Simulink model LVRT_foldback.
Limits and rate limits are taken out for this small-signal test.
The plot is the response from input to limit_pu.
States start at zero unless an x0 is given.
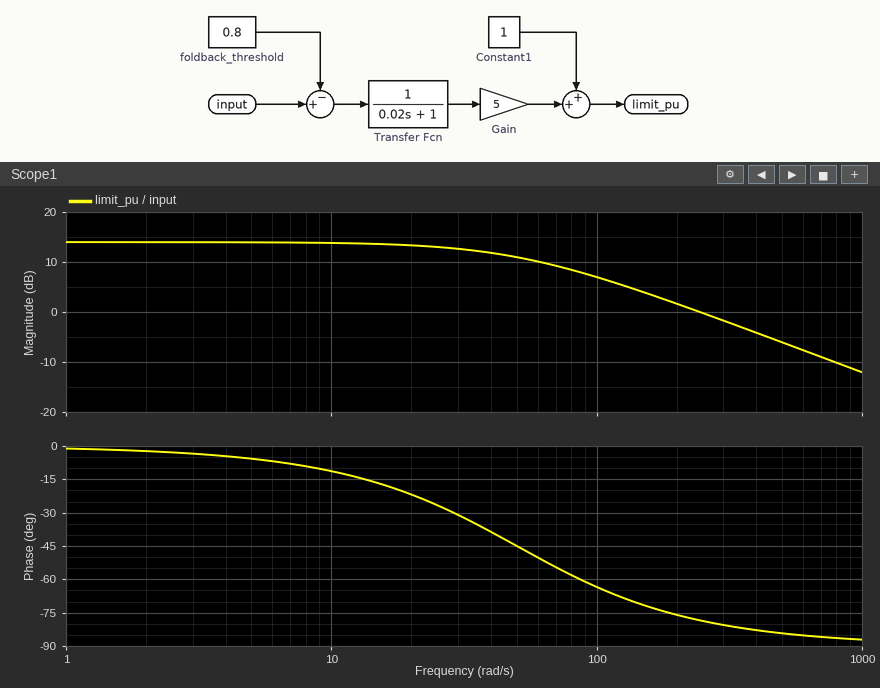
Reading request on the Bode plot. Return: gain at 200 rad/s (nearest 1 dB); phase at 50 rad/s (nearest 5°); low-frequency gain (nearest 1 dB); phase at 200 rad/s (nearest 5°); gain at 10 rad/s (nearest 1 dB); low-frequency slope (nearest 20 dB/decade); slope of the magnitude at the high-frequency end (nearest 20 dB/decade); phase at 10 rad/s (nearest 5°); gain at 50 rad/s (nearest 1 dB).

2 dB
-45°
14 dB
-75°
14 dB
0 dB/decade
-20 dB/decade
-10°
11 dB
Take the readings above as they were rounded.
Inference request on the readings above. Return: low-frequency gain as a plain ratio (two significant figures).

5.0
